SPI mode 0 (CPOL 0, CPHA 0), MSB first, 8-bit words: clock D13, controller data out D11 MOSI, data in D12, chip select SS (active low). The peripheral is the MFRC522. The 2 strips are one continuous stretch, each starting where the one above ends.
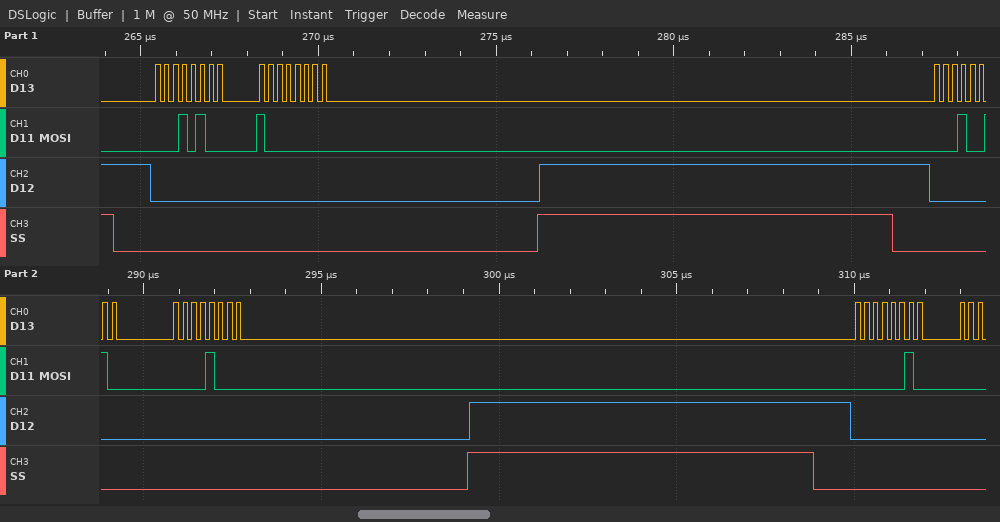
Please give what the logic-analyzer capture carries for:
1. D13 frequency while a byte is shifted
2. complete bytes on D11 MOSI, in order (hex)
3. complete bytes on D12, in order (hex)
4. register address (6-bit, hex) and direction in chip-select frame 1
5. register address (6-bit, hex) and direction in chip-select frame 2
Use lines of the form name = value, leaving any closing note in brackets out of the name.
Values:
D13 frequency while a byte is shifted = 4 MHz
complete bytes on D11 MOSI, in order = 14 80 12 08 02
complete bytes on D12, in order = 00 00 00 00 00
register address (6-bit, hex) and direction in chip-select frame 1 = 0x0A write
register address (6-bit, hex) and direction in chip-select frame 2 = 0x09 write
